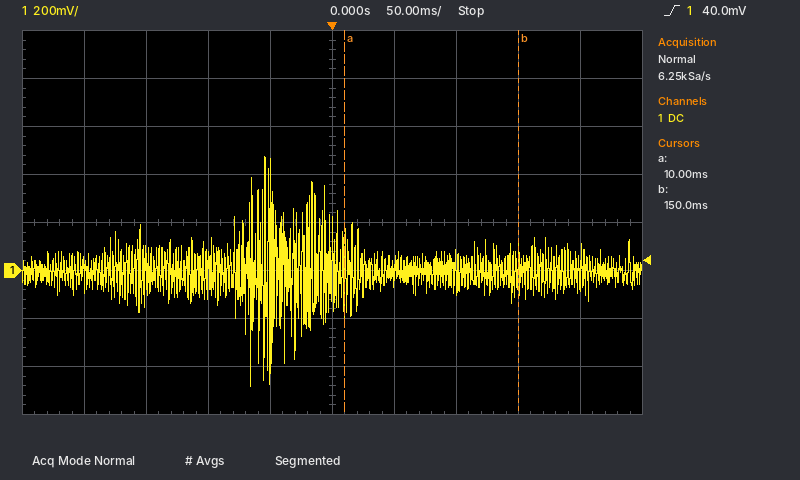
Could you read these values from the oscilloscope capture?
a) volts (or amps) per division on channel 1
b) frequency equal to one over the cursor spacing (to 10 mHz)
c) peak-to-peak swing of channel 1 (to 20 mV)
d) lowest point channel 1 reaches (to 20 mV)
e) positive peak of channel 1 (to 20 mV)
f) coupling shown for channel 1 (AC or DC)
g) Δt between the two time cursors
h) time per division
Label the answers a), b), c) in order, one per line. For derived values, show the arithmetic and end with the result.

a) 200 mV
b) 1 / 140 ms ≈ 7.14 Hz
c) 480 mV − (-480 mV) = 960 mV
d) -480 mV
e) 480 mV
f) DC
g) 150 ms − (10 ms) = 140 ms
h) 50 ms
